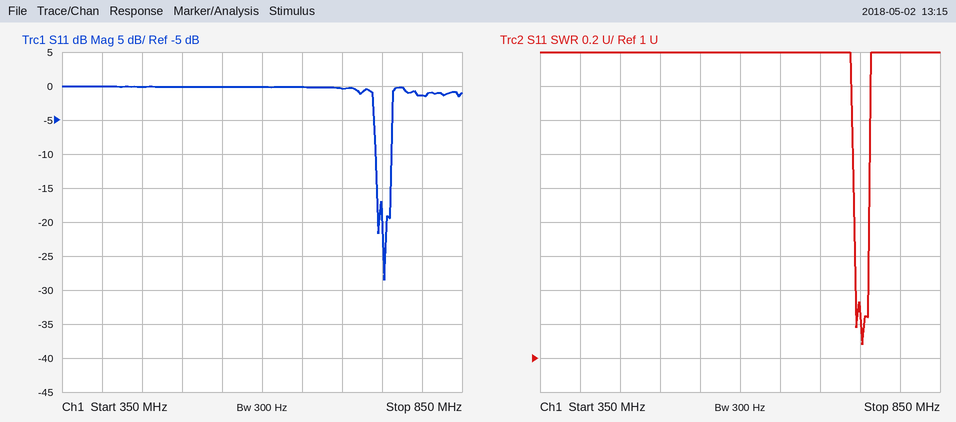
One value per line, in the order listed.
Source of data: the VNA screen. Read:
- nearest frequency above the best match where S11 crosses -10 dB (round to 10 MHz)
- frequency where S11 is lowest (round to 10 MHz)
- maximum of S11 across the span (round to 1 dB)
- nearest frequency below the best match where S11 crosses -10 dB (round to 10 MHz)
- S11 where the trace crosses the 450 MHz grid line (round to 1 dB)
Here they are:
760 MHz
750 MHz
0 dB
740 MHz
0 dB
